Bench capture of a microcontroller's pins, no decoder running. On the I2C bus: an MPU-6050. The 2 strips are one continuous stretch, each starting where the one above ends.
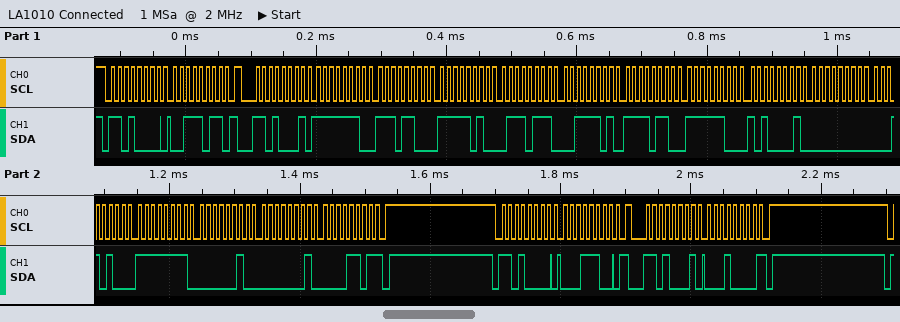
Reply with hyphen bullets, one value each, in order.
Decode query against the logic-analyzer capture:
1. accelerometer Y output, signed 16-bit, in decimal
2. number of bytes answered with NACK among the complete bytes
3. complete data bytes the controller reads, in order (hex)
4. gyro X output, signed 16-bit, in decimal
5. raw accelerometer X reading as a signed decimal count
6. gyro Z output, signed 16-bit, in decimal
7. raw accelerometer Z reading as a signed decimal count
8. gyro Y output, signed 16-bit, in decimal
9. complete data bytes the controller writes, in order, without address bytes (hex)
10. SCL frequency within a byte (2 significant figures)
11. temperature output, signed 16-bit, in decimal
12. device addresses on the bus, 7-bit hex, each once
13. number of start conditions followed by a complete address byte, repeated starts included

- -1417
- 2
- FE EC FA 77 3D F6 FC A1 00 14 FF 02 01 0D 10
- 20
- -276
- 269
- 15862
- -254
- 3B 1C
- 100 kHz
- -863
- 0x68
- 4
